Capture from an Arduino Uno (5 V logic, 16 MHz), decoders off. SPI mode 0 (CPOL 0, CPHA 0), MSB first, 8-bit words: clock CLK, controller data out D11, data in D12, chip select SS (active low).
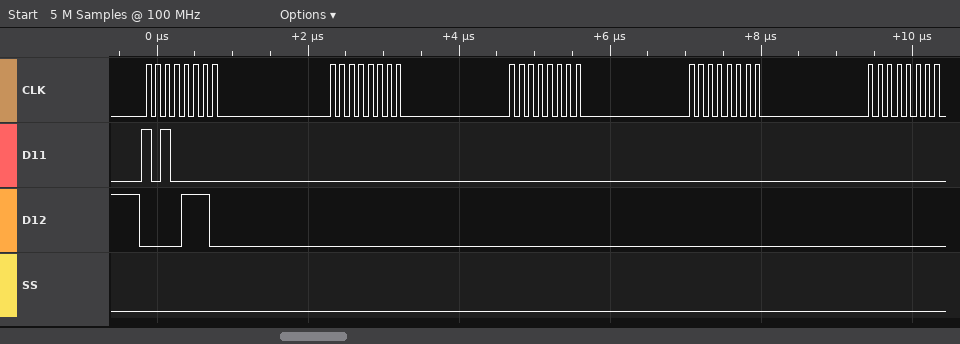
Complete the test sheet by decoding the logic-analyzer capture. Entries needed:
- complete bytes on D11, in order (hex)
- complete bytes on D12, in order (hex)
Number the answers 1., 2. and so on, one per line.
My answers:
1. A0 00 00 00 00
2. 0E 00 00 00 00
